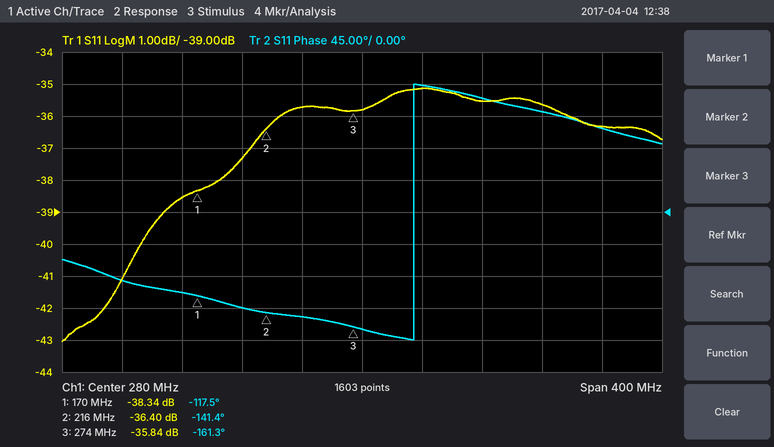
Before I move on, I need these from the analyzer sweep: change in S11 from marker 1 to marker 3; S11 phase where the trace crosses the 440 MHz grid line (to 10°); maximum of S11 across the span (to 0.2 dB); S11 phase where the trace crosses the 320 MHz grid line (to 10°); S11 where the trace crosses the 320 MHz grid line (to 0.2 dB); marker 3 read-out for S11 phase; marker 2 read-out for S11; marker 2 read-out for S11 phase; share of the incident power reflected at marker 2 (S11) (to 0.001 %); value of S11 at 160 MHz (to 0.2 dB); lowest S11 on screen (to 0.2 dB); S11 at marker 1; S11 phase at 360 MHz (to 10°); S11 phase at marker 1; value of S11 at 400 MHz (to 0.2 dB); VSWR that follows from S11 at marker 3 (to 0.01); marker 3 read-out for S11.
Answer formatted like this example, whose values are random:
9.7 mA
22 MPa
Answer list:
2.50 dB
120°
-35.2 dB
180°
-35.2 dB
-161.3°
-36.40 dB
-141.4°
0.023 %
-38.6 dB
-43.0 dB
-38.34 dB
160°
-117.5°
-35.6 dB
1.03
-35.84 dB
